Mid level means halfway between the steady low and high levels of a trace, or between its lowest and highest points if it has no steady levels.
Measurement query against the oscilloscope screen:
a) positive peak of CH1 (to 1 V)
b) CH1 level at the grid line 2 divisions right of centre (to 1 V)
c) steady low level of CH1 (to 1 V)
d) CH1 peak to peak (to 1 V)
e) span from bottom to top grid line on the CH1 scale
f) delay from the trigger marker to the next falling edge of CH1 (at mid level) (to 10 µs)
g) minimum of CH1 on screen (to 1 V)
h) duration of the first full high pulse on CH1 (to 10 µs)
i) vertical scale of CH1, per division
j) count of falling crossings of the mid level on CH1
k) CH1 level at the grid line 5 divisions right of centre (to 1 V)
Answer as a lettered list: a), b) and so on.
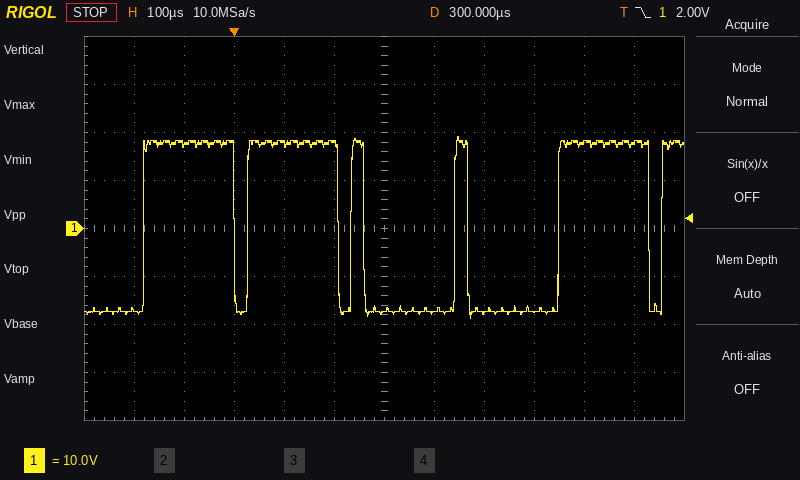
a) 19 V
b) -18 V
c) -17 V
d) 38 V
e) 80 V
f) 210 µs
g) -19 V
h) 180 µs
i) 10 V
j) 5
k) 18 V
